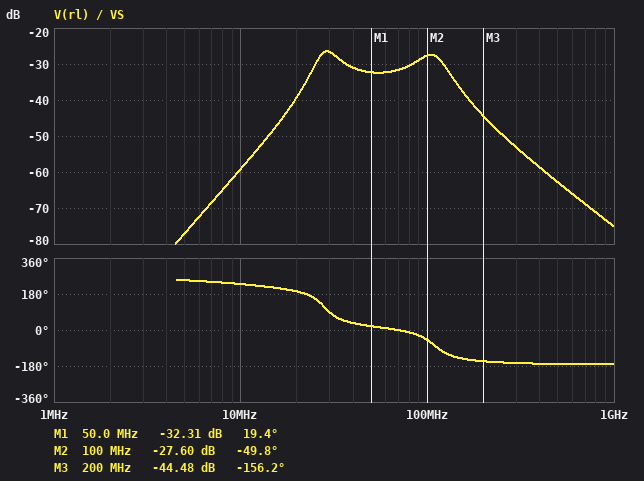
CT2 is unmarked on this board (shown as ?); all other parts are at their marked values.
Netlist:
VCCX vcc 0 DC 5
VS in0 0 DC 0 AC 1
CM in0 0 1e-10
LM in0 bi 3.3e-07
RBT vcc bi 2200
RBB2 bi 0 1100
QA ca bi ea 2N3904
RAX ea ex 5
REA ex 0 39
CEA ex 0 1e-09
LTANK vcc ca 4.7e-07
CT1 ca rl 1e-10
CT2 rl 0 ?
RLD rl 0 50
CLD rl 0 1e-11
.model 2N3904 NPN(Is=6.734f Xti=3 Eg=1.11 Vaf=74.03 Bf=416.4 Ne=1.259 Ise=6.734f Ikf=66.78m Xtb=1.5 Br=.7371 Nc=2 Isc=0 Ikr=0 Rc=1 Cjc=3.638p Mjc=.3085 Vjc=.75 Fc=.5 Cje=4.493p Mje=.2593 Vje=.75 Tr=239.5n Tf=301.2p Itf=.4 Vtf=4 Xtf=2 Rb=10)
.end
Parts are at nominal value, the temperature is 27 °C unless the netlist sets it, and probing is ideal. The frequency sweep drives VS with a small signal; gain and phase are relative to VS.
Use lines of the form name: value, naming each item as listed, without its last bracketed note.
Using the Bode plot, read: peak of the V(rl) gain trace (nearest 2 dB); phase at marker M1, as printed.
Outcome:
peak of the V(rl) gain trace: -26 dB
phase at marker M1, as printed: 19.4 deg
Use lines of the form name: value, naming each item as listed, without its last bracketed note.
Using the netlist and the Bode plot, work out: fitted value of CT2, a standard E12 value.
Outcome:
fitted value of CT2, a standard E12 value: 120 pF
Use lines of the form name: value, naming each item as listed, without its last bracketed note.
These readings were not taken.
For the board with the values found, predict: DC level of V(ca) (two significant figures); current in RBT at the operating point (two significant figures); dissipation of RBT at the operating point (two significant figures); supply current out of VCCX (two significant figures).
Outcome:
DC level of V(ca): 5.0 V
current in RBT at the operating point: 2.3 mA
dissipation of RBT at the operating point: 11 mW
supply current out of VCCX: 2.3 mA
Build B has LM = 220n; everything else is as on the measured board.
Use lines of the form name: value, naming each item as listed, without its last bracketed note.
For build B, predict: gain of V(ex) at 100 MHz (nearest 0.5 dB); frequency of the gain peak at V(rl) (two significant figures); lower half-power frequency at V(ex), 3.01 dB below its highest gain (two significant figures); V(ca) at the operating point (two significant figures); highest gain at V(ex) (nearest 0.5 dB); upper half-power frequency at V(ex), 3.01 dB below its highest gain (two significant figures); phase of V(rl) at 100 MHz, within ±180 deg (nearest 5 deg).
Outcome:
gain of V(ex) at 100 MHz: -41.0 dB
frequency of the gain peak at V(rl): 130 MHz
lower half-power frequency at V(ex), 3.01 dB below its highest gain: 110 MHz
V(ca) at the operating point: 5.0 V
highest gain at V(ex): -37.0 dB
upper half-power frequency at V(ex), 3.01 dB below its highest gain: 150 MHz
phase of V(rl) at 100 MHz, within ±180 deg: -15 deg
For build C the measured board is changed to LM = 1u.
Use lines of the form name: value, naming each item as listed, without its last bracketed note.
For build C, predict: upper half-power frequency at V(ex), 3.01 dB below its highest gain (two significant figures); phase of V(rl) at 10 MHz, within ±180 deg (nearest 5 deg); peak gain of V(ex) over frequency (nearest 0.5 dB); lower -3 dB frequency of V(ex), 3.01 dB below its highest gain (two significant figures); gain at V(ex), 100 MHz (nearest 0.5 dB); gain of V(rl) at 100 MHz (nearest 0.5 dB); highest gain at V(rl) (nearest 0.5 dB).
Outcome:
upper half-power frequency at V(ex), 3.01 dB below its highest gain: 74 MHz
phase of V(rl) at 10 MHz, within ±180 deg: -135 deg
peak gain of V(ex) over frequency: -42.0 dB
lower -3 dB frequency of V(ex), 3.01 dB below its highest gain: 34 MHz
gain at V(ex), 100 MHz: -52.0 dB
gain of V(rl) at 100 MHz: -41.5 dB
highest gain at V(rl): -25.5 dB
